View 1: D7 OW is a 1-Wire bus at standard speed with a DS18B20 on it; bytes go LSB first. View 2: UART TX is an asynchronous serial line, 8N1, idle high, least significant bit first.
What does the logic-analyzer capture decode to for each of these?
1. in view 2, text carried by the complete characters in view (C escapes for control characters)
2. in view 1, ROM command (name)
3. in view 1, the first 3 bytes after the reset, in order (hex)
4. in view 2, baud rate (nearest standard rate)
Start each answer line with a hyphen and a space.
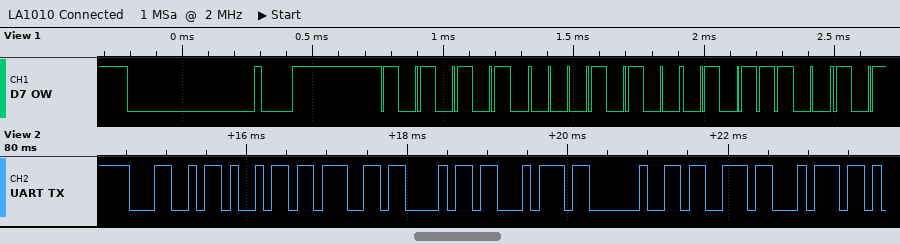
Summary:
- "Light st"
- Match ROM
- 55 28 3A
- 9600 baud
